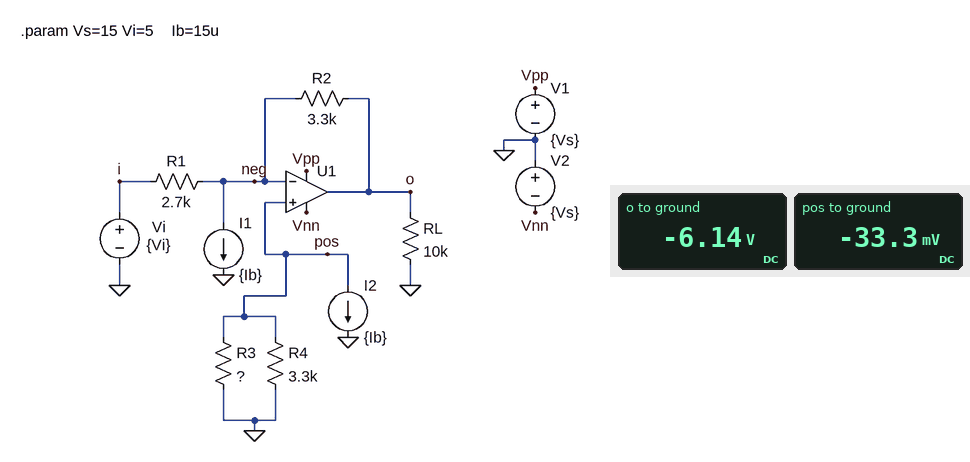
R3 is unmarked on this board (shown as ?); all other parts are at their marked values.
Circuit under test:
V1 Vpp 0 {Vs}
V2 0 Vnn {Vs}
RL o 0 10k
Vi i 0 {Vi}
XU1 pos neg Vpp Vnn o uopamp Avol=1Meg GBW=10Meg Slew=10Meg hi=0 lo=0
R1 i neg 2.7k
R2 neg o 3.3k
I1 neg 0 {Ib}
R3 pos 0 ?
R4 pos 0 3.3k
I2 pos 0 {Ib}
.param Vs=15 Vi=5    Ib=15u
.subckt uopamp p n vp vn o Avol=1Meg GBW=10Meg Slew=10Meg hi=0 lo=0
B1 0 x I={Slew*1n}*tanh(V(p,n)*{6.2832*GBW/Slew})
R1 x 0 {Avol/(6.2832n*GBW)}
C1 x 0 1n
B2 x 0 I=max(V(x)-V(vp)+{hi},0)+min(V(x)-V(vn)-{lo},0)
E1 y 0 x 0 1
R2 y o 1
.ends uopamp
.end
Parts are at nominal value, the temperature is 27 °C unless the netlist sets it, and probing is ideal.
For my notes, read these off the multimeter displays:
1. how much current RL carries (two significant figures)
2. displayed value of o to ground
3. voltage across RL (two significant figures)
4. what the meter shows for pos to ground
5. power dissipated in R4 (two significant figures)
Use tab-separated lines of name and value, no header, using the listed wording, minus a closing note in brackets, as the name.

how much current RL carries	610 µA
displayed value of o to ground	-6.14 V
voltage across RL	6.1 V
what the meter shows for pos to ground	-33.3 mV
power dissipated in R4	340 nW
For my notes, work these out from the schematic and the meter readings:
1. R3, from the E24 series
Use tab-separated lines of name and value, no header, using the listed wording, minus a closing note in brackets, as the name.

R3, from the E24 series	6.8 kΩ
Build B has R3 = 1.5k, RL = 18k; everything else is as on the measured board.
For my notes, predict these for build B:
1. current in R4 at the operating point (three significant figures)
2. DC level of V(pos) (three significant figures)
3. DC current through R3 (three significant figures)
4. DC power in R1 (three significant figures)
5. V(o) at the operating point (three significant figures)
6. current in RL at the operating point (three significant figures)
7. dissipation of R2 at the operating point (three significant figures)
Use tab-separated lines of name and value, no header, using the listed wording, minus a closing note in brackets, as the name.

current in R4 at the operating point	4.69 µA
DC level of V(pos)	-15.5 mV
DC current through R3	10.3 µA
DC power in R1	9.32 mW
V(o) at the operating point	-6.10 V
current in RL at the operating point	339 µA
dissipation of R2 at the operating point	11.2 mW
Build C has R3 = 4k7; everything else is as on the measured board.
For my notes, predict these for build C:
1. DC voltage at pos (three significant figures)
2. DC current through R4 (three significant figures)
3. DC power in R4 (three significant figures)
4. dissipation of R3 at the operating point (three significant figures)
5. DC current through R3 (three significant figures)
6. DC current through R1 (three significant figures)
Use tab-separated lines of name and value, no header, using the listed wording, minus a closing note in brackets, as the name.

DC voltage at pos	-29.1 mV
DC current through R4	8.81 µA
DC power in R4	256 nW
dissipation of R3 at the operating point	180 nW
DC current through R3	6.19 µA
DC current through R1	1.86 mA
